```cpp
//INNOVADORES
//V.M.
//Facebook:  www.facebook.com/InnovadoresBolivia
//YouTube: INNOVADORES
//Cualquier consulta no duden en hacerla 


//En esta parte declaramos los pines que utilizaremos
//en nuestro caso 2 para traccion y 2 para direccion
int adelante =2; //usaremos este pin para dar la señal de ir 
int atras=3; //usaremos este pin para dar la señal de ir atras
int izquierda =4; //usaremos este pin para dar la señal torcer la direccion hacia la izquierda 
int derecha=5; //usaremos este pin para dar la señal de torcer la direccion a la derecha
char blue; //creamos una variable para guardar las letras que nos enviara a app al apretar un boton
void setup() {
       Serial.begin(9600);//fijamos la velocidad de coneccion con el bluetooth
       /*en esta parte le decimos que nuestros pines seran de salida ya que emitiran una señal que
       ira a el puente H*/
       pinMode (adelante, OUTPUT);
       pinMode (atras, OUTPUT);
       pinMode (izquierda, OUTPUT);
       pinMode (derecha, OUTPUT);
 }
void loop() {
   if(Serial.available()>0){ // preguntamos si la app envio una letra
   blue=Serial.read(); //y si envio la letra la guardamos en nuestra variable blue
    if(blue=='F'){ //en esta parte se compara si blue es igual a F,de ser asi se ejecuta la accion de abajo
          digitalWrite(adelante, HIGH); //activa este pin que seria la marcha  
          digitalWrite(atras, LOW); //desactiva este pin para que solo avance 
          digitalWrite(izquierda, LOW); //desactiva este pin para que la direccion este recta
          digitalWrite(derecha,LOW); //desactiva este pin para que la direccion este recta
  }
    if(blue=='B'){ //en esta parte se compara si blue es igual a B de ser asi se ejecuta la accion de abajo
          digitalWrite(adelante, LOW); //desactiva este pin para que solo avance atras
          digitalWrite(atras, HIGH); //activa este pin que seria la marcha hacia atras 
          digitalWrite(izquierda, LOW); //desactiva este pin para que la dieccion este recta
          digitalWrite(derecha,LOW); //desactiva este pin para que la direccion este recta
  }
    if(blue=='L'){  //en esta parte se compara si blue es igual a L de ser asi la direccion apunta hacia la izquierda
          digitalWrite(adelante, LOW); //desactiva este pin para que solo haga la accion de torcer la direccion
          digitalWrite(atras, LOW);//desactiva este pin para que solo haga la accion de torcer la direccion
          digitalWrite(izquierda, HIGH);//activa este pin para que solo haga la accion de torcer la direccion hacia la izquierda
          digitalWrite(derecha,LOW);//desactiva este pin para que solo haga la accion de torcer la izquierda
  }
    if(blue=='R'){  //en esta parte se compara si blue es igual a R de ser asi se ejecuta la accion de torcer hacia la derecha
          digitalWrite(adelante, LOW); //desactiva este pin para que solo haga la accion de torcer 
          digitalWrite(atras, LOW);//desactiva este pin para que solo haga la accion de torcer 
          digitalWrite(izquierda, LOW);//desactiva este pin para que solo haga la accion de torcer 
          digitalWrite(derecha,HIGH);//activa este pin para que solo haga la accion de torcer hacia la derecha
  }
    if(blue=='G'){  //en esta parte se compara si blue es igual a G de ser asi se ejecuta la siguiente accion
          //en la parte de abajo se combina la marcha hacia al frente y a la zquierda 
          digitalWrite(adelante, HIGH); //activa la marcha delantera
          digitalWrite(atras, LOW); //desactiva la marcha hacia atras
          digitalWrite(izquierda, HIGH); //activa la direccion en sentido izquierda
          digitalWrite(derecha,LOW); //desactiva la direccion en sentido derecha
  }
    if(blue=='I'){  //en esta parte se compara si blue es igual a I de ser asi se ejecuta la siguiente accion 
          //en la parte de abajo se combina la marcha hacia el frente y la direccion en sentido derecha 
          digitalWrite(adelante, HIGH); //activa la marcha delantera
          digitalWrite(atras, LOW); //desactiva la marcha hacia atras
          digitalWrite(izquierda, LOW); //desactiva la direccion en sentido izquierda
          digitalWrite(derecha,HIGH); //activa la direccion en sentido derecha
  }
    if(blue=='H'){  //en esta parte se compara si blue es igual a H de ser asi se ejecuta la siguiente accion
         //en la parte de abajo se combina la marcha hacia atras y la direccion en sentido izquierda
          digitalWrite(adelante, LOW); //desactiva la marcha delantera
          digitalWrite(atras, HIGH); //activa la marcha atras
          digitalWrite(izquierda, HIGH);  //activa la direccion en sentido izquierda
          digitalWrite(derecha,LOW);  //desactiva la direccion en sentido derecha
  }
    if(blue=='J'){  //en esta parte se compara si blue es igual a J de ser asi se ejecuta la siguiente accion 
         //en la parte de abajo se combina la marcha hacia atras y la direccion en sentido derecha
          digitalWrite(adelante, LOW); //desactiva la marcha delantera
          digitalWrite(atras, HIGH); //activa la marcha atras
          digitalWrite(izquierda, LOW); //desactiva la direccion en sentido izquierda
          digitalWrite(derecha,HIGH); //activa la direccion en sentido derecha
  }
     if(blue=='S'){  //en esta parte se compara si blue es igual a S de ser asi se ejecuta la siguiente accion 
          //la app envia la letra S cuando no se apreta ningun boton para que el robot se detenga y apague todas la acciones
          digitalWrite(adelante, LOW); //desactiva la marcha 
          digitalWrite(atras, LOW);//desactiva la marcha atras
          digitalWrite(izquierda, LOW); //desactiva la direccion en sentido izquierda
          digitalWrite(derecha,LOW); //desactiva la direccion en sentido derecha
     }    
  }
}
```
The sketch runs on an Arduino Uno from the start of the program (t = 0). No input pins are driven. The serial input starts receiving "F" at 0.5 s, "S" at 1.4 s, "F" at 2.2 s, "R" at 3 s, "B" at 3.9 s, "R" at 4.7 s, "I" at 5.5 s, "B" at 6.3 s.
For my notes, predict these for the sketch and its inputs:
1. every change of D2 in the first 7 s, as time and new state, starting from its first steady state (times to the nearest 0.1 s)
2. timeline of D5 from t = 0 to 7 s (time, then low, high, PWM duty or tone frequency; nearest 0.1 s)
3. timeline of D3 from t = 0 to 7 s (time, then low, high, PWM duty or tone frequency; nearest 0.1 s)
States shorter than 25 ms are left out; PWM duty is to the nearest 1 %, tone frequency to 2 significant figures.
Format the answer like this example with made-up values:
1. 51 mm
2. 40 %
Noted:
1. 0 s low; 0.5 s high; 1.4 s low; 2.2 s high; 3 s low; 5.5 s high; 6.3 s low
2. 0 s low; 3 s high; 3.9 s low; 4.7 s high; 6.3 s low
3. 0 s low; 3.9 s high; 4.7 s low; 6.3 s high
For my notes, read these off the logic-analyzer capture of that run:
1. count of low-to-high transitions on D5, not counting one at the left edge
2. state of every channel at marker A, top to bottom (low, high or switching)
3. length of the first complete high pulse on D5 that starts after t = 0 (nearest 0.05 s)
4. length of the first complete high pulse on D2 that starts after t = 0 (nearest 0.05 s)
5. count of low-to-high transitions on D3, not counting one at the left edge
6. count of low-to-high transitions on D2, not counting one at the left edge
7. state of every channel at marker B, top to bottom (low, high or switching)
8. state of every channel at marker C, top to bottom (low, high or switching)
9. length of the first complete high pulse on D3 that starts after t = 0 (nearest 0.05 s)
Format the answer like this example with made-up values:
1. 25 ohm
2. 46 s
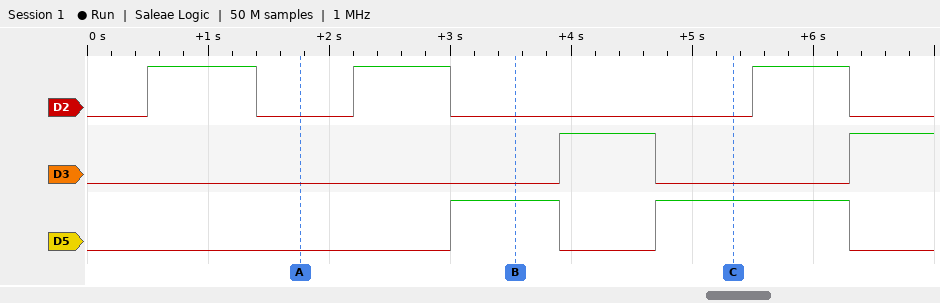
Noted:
1. 2
2. D2 low, D3 low, D5 low
3. 0.90 s
4. 0.90 s
5. 2
6. 3
7. D2 low, D3 low, D5 high
8. D2 low, D3 low, D5 high
9. 0.80 s
